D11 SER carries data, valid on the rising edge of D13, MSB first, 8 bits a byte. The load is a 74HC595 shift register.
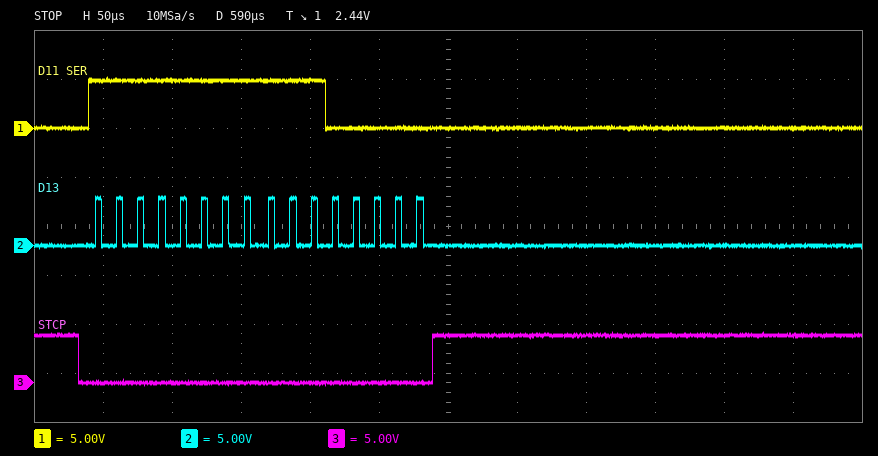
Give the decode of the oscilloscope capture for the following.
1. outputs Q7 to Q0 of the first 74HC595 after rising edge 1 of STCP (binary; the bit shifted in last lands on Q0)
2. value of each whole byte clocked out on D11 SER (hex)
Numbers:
11100000
FF E0
